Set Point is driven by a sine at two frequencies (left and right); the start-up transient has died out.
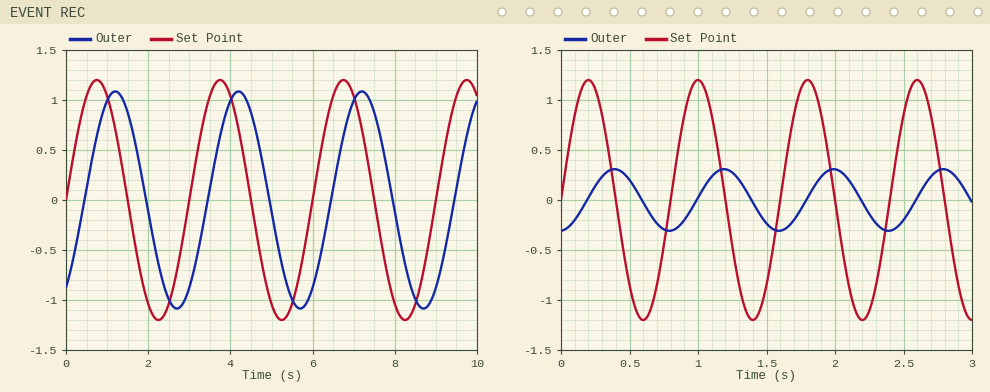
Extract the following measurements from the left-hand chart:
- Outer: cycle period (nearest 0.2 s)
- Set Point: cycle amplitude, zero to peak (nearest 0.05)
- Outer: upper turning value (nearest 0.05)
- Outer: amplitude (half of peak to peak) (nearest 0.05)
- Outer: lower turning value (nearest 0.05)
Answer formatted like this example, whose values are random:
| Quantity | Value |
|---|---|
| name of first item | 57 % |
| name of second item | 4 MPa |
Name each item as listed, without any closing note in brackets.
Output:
| Quantity | Value |
|---|---|
| Outer: cycle period | 3.0 s |
| Set Point: cycle amplitude, zero to peak | 1.20 |
| Outer: upper turning value | 1.10 |
| Outer: amplitude (half of peak to peak) | 1.10 |
| Outer: lower turning value | -1.10 |
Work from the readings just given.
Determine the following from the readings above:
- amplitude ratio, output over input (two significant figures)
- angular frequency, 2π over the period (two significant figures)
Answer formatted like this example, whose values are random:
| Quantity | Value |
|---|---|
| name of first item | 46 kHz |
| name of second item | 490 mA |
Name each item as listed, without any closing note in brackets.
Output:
| Quantity | Value |
|---|---|
| amplitude ratio, output over input | 0.92 |
| angular frequency, 2π over the period | 2.1 rad/s |
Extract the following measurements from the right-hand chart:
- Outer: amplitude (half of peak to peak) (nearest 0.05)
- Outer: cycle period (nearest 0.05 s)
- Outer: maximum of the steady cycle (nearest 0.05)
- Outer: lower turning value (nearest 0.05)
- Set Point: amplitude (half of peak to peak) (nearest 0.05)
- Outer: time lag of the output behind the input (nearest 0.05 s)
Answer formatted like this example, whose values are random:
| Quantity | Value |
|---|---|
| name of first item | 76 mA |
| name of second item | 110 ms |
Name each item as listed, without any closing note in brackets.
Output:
| Quantity | Value |
|---|---|
| Outer: amplitude (half of peak to peak) | 0.30 |
| Outer: cycle period | 0.80 s |
| Outer: maximum of the steady cycle | 0.30 |
| Outer: lower turning value | -0.30 |
| Set Point: amplitude (half of peak to peak) | 1.20 |
| Outer: time lag of the output behind the input | 0.20 s |
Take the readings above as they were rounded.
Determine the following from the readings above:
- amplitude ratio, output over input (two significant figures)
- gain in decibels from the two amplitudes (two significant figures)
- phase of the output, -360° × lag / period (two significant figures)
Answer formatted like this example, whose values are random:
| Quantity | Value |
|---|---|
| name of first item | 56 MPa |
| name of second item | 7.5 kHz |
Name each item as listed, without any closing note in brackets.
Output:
| Quantity | Value |
|---|---|
| amplitude ratio, output over input | 0.25 |
| gain in decibels from the two amplitudes | -12 dB |
| phase of the output, -360° × lag / period | -90° |
